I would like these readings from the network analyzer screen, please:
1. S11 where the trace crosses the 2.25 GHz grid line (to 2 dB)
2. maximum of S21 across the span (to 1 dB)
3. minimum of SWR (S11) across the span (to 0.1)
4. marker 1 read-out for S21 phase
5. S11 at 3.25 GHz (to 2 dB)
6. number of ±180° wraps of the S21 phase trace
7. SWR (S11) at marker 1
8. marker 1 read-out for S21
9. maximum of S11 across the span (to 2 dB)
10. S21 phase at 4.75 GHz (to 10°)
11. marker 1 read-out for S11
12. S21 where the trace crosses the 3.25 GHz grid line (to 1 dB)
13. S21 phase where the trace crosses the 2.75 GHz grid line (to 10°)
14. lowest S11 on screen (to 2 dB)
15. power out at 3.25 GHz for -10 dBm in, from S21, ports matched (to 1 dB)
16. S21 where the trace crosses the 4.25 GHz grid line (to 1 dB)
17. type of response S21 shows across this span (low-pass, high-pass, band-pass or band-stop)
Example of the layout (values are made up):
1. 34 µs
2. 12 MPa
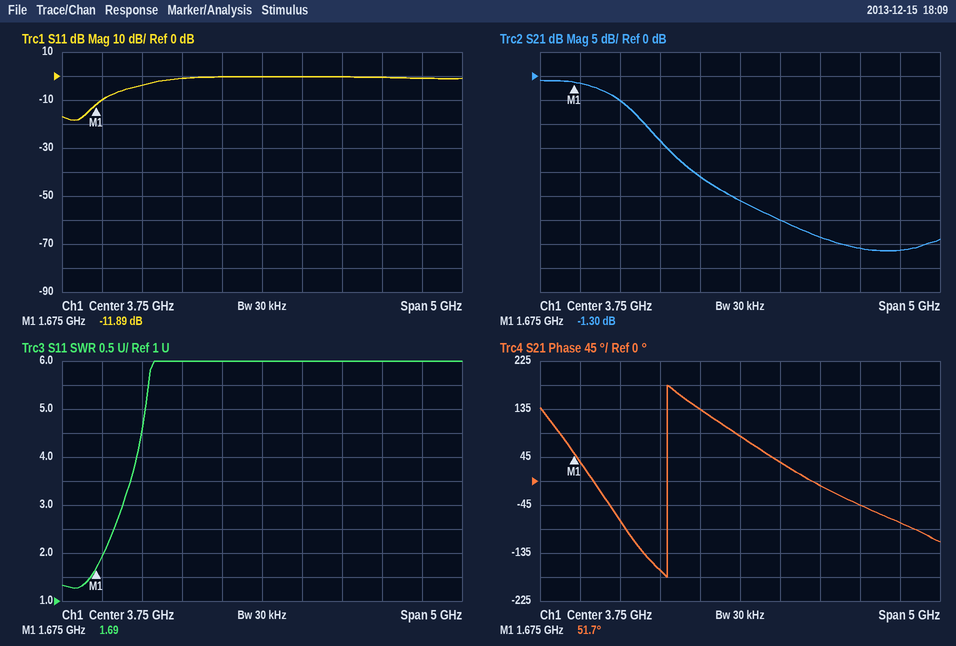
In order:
1. -4 dB
2. -1 dB
3. 1.3
4. 51.7°
5. 0 dB
6. 1
7. 1.69
8. -1.30 dB
9. 0 dB
10. -10°
11. -11.89 dB
12. -21 dB
13. -170°
14. -18 dB
15. -31 dBm
16. -30 dB
17. low-pass
